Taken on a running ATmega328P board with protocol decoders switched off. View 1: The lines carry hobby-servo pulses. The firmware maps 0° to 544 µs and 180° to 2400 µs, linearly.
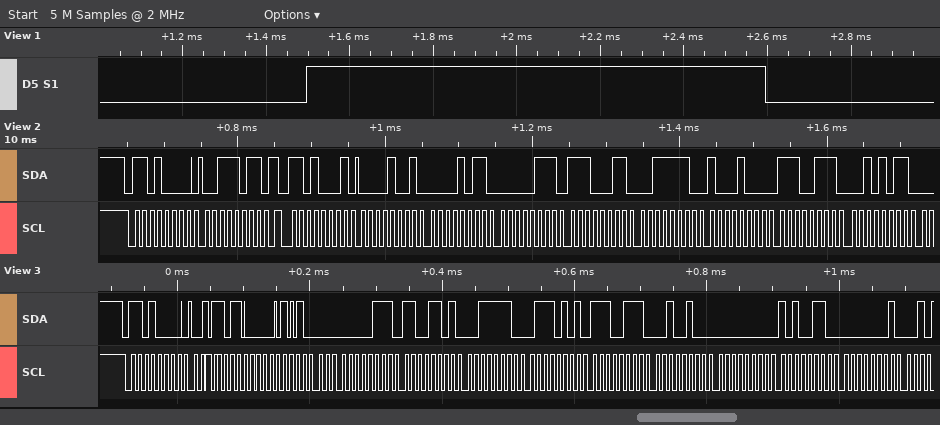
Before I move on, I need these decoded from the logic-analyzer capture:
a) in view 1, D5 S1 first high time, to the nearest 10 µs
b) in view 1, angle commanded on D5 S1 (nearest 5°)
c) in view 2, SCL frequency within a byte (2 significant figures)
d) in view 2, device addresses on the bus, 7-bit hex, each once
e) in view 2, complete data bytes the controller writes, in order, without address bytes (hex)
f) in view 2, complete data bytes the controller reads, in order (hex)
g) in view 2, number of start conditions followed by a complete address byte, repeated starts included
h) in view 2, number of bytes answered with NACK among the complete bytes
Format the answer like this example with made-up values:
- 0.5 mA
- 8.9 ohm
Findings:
- 1100 µs
- 55°
- 100 kHz
- 0x68
- 3B
- 09 0B 07 E3 3E 88 E7 2B
- 2
- 0
